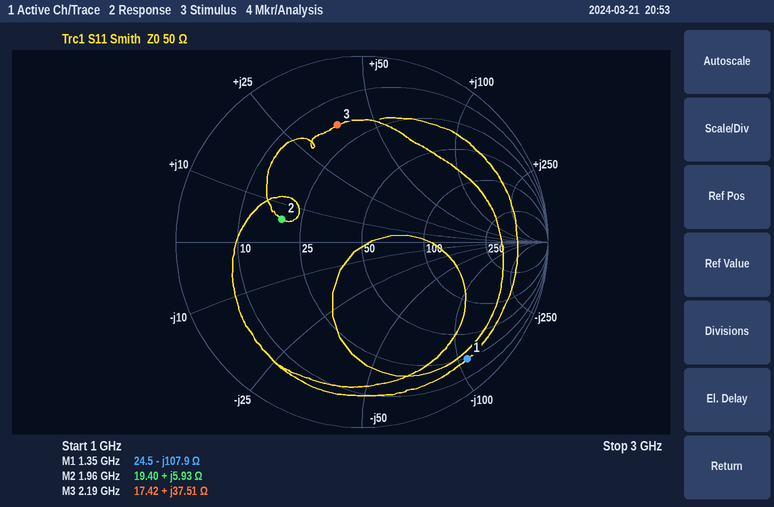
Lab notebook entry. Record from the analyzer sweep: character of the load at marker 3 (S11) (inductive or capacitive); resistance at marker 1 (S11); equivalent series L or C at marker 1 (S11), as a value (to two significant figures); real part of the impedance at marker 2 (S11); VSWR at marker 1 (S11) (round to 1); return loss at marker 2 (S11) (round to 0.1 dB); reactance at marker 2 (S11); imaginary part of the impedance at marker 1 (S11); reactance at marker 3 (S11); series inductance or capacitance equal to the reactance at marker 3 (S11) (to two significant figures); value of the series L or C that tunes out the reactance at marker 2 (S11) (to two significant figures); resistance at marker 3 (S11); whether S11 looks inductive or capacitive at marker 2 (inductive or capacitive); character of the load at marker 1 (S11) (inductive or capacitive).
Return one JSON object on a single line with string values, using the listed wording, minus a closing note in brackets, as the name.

{"character of the load at marker 3 (S11)": "inductive", "resistance at marker 1": "24.5 Ω", "equivalent series L or C at marker 1 (S11), as a value": "1.1 pF", "real part of the impedance at marker 2": "19.40 Ω", "VSWR at marker 1 (S11)": "12", "return loss at marker 2 (S11)": "7.0 dB", "reactance at marker 2": "+5.93 Ω", "imaginary part of the impedance at marker 1": "-107.9 Ω", "reactance at marker 3": "+37.51 Ω", "series inductance or capacitance equal to the reactance at marker 3 (S11)": "2.7 nH", "value of the series L or C that tunes out the reactance at marker 2 (S11)": "14 pF", "resistance at marker 3": "17.42 Ω", "whether S11 looks inductive or capacitive at marker 2": "inductive", "character of the load at marker 1 (S11)": "capacitive"}
